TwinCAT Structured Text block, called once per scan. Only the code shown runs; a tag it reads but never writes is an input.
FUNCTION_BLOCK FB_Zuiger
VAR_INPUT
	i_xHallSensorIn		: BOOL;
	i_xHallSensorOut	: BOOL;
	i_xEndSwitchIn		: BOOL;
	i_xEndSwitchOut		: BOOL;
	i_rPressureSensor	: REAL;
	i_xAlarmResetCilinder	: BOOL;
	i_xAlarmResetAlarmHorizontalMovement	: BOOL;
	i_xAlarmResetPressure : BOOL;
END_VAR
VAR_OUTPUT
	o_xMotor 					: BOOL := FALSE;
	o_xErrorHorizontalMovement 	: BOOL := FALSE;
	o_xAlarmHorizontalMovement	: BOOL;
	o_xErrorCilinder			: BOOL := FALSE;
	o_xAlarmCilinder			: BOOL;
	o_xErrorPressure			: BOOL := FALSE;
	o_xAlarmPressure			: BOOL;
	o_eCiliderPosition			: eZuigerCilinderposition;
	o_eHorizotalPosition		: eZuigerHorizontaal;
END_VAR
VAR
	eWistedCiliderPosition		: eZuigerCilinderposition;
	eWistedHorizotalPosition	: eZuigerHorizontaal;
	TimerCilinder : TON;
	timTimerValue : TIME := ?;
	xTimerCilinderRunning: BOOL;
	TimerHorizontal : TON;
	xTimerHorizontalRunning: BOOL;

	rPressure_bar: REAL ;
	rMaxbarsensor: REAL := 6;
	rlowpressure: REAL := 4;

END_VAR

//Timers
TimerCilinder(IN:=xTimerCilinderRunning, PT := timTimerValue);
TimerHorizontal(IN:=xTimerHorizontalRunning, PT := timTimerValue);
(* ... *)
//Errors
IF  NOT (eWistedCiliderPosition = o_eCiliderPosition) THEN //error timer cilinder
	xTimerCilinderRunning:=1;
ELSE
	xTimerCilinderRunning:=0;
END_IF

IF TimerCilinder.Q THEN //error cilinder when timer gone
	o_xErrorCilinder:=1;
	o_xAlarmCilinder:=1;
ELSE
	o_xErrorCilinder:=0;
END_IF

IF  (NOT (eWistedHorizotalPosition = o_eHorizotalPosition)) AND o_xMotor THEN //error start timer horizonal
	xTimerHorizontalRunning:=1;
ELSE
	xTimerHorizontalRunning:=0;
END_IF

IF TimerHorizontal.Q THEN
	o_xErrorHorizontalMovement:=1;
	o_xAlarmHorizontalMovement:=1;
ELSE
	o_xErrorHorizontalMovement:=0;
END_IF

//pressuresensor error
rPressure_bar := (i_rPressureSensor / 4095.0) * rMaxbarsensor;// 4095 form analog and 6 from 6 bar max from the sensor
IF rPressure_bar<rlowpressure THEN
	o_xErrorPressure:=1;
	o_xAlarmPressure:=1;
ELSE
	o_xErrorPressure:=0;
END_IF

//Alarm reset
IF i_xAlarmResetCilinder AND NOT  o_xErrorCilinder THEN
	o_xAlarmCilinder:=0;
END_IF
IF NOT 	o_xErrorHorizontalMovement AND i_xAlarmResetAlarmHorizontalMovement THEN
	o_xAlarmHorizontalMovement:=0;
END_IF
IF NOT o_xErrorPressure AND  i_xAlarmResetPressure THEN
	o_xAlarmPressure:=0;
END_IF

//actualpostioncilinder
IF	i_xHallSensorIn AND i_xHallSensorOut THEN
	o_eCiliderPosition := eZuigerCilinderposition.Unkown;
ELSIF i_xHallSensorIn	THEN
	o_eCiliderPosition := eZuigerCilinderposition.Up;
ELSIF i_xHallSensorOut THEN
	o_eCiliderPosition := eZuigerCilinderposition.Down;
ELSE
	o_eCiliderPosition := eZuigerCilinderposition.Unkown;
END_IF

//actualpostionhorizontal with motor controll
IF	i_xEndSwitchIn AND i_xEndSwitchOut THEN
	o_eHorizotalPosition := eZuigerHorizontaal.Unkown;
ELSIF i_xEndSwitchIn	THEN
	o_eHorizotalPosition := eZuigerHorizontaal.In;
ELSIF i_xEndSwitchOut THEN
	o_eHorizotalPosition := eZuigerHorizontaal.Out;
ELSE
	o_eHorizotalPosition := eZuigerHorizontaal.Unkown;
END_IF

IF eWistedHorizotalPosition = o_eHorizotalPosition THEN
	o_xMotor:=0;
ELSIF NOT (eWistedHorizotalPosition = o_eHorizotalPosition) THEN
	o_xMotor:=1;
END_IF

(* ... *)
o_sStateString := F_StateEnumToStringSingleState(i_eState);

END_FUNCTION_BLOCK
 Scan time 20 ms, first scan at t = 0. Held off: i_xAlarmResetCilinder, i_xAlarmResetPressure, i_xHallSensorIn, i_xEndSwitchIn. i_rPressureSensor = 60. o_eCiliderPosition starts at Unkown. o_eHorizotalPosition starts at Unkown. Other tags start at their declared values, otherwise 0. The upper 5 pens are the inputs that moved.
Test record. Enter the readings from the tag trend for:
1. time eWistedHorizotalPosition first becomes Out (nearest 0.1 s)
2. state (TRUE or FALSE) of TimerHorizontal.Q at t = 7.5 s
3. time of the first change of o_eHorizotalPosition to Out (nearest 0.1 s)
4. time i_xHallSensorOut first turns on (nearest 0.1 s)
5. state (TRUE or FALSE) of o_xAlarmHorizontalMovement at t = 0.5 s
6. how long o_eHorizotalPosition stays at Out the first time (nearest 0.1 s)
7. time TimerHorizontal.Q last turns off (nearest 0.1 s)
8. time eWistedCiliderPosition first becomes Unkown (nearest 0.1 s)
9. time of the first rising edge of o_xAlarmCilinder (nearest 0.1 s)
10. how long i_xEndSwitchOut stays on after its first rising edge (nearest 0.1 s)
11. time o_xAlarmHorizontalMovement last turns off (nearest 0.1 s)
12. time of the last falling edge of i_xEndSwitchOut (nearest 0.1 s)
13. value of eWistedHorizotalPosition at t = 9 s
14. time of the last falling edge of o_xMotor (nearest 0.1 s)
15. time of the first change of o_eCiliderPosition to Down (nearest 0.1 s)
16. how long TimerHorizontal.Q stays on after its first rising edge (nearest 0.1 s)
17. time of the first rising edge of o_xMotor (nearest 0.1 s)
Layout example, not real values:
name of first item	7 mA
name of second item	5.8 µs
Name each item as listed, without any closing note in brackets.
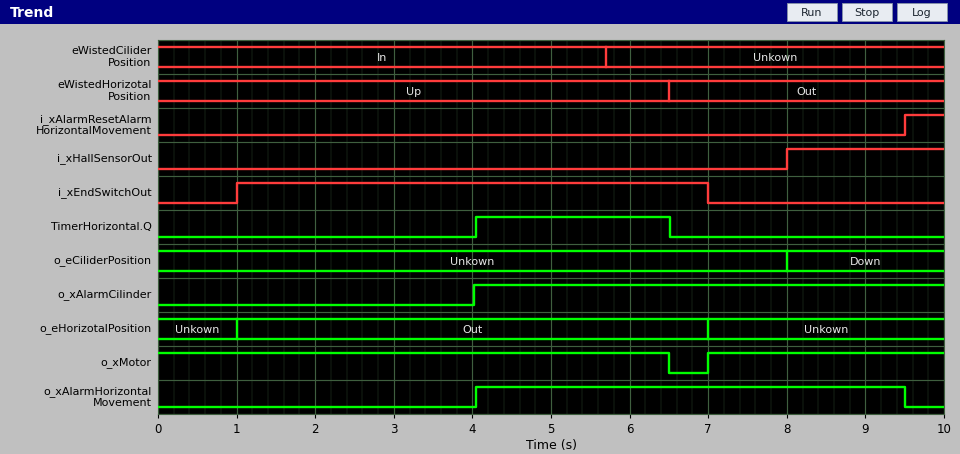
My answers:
time eWistedHorizotalPosition first becomes Out	6.5 s
state (TRUE or FALSE) of TimerHorizontal.Q at t = 7.5 s	FALSE
time of the first change of o_eHorizotalPosition to Out	1.0 s
time i_xHallSensorOut first turns on	8.0 s
state (TRUE or FALSE) of o_xAlarmHorizontalMovement at t = 0.5 s	FALSE
how long o_eHorizotalPosition stays at Out the first time	6.0 s
time TimerHorizontal.Q last turns off	6.5 s
time eWistedCiliderPosition first becomes Unkown	5.7 s
time of the first rising edge of o_xAlarmCilinder	4.0 s
how long i_xEndSwitchOut stays on after its first rising edge	6.0 s
time o_xAlarmHorizontalMovement last turns off	9.5 s
time of the last falling edge of i_xEndSwitchOut	7.0 s
value of eWistedHorizotalPosition at t = 9 s	Out
time of the last falling edge of o_xMotor	6.5 s
time of the first change of o_eCiliderPosition to Down	8.0 s
how long TimerHorizontal.Q stays on after its first rising edge	2.5 s
time of the first rising edge of o_xMotor	7.0 s
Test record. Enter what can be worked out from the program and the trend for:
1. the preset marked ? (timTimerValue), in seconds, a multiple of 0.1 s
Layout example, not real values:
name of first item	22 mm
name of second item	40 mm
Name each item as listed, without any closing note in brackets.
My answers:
the preset marked ? (timTimerValue), in seconds, a multiple of 0.1 s	4.0 s
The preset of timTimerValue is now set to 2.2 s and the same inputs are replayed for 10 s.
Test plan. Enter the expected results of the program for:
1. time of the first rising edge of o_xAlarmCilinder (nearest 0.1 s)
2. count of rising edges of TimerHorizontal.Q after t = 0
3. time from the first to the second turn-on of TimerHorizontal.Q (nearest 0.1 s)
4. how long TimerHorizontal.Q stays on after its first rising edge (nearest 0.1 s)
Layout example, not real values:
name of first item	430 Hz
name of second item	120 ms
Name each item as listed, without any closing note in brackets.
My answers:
time of the first rising edge of o_xAlarmCilinder	2.2 s
count of rising edges of TimerHorizontal.Q after t = 0	2
time from the first to the second turn-on of TimerHorizontal.Q	7.0 s
how long TimerHorizontal.Q stays on after its first rising edge	4.3 s
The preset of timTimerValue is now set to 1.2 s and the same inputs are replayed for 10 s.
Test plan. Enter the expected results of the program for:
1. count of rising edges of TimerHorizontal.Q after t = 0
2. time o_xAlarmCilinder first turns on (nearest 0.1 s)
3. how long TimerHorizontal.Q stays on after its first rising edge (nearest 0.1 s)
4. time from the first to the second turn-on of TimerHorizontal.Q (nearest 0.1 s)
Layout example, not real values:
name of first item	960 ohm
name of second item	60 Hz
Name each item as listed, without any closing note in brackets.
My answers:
count of rising edges of TimerHorizontal.Q after t = 0	2
time o_xAlarmCilinder first turns on	1.2 s
how long TimerHorizontal.Q stays on after its first rising edge	5.3 s
time from the first to the second turn-on of TimerHorizontal.Q	7.0 s
